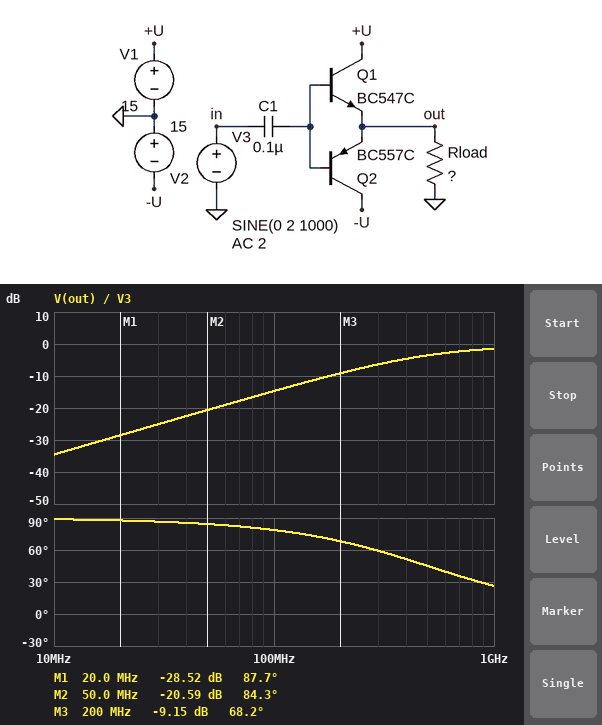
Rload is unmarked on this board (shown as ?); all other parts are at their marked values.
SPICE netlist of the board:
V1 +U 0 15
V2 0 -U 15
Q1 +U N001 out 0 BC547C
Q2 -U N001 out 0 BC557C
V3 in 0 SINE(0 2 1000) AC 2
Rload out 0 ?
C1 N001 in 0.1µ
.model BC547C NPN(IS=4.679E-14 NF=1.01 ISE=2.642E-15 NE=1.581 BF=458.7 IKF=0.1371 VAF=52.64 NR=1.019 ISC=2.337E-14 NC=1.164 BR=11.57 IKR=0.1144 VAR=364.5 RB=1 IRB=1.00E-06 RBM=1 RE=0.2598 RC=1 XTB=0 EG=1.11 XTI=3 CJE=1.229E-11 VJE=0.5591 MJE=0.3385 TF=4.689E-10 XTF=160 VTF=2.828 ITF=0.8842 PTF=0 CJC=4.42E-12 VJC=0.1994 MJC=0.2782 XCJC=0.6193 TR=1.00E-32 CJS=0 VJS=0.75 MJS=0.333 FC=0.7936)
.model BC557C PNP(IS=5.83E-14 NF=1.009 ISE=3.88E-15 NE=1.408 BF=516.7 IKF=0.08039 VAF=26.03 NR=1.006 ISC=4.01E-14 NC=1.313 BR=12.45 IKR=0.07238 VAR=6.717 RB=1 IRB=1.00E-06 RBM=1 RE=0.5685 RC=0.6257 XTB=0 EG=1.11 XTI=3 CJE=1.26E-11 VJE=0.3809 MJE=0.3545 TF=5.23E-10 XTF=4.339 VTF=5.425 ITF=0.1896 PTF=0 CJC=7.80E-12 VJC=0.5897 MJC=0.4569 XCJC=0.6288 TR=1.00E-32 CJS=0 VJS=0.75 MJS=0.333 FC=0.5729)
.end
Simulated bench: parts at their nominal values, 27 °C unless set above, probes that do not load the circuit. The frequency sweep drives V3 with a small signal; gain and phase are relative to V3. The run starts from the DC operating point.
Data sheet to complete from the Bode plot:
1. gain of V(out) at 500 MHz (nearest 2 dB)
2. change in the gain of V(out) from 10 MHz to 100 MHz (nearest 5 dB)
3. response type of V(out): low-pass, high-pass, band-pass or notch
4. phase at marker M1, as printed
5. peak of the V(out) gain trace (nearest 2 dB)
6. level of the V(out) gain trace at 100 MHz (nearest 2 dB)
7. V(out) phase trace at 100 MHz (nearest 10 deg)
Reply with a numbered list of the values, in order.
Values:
1. -4 dB
2. 20 dB
3. high-pass
4. 87.7 deg
5. -2 dB
6. -14 dB
7. 80 deg
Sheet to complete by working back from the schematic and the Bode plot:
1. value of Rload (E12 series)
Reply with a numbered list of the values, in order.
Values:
1. 12 Ω
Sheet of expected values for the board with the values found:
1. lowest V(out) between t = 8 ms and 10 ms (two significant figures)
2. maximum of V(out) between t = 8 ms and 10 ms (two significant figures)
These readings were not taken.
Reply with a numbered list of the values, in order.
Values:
1. -1.2 V
2. 1.2 V
